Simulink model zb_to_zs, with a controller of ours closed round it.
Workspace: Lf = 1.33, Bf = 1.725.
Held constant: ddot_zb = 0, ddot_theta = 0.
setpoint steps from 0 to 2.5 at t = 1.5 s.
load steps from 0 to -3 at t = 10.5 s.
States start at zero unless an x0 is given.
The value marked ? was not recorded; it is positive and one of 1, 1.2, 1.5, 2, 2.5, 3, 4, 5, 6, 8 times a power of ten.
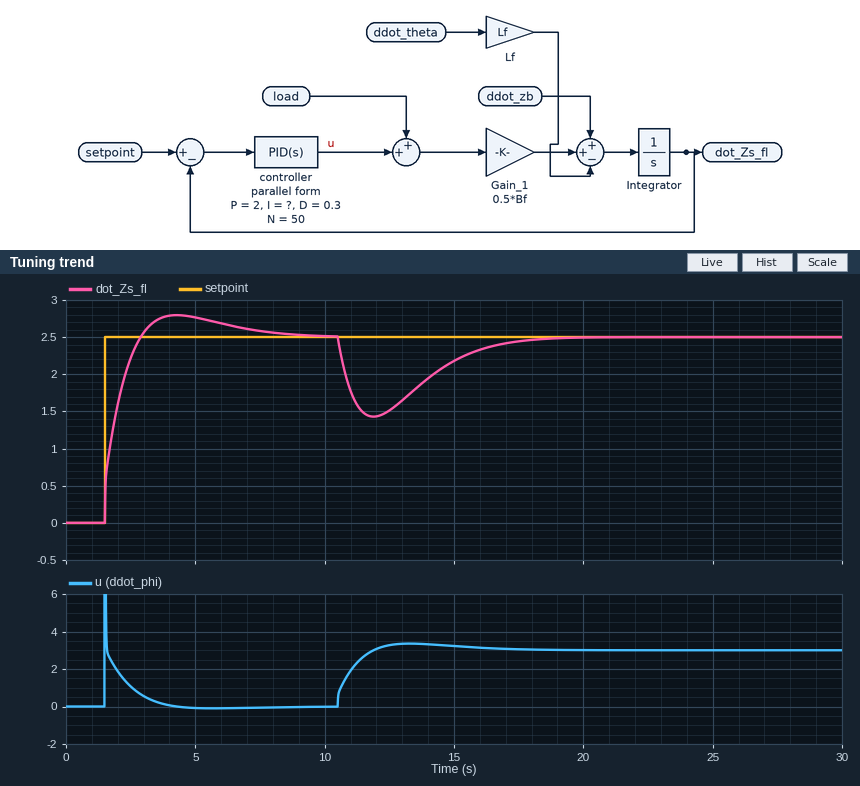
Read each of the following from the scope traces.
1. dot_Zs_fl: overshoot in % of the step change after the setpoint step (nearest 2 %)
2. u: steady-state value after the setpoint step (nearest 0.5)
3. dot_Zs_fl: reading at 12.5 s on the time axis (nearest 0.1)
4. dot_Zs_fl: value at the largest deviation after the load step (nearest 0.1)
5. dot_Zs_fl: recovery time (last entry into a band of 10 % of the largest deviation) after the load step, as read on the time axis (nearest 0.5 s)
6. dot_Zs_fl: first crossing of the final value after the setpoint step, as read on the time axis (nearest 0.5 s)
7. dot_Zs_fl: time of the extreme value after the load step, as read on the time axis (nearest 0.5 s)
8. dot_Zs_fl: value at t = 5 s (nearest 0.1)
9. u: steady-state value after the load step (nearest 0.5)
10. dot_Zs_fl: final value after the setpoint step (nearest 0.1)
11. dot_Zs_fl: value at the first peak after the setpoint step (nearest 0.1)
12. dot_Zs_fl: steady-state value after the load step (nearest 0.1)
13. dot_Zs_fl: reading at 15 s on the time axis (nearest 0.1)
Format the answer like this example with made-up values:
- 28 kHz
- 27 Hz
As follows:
- 12 %
- 0.0
- 1.5
- 1.4
- 16.5 s
- 3.0 s
- 12.0 s
- 2.8
- 3.0
- 2.5
- 2.8
- 2.5
- 2.2
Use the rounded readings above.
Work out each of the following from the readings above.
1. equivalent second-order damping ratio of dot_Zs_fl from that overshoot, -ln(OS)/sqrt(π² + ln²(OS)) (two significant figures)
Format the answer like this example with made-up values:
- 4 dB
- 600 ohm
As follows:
- 0.56
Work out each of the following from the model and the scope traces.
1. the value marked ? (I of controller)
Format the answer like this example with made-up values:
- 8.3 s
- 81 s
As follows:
- 0.8
